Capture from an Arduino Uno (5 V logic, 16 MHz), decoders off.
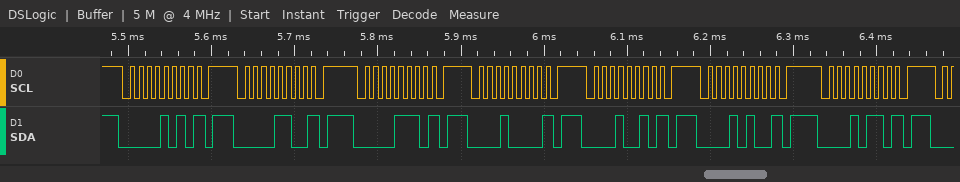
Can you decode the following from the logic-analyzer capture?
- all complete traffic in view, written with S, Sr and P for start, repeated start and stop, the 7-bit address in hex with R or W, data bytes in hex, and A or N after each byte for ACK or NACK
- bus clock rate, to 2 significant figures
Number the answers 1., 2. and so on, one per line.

1. S 05W N P S 06W N P S 07W N P S 08W N P S 09W N P S 0AW N P S 0BW N P
2. 100 kHz
